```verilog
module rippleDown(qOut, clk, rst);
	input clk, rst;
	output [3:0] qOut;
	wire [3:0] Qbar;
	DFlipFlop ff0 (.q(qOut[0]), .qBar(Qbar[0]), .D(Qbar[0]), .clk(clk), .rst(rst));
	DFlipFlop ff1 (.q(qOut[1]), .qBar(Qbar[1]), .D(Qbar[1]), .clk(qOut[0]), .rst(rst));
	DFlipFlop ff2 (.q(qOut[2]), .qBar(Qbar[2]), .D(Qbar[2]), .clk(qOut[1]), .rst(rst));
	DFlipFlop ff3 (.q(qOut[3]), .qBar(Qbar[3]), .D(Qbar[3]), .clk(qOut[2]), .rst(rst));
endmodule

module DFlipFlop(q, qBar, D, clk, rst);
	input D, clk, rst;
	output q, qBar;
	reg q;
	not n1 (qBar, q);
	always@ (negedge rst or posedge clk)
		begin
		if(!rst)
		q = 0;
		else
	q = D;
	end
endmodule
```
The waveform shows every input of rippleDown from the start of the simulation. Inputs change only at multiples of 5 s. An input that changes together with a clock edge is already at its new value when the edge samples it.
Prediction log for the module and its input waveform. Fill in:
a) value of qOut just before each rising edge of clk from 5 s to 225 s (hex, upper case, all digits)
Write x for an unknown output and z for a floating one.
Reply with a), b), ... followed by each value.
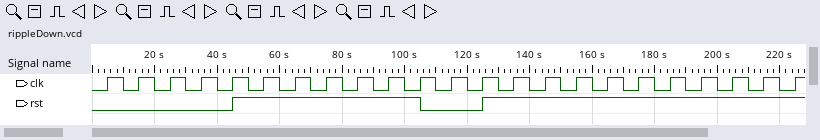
a) 0, 0, 0, 0, 0, F, E, D, C, B, A, 0, 0, F, E, D, C, B, A, 9, 8, 7, 6
